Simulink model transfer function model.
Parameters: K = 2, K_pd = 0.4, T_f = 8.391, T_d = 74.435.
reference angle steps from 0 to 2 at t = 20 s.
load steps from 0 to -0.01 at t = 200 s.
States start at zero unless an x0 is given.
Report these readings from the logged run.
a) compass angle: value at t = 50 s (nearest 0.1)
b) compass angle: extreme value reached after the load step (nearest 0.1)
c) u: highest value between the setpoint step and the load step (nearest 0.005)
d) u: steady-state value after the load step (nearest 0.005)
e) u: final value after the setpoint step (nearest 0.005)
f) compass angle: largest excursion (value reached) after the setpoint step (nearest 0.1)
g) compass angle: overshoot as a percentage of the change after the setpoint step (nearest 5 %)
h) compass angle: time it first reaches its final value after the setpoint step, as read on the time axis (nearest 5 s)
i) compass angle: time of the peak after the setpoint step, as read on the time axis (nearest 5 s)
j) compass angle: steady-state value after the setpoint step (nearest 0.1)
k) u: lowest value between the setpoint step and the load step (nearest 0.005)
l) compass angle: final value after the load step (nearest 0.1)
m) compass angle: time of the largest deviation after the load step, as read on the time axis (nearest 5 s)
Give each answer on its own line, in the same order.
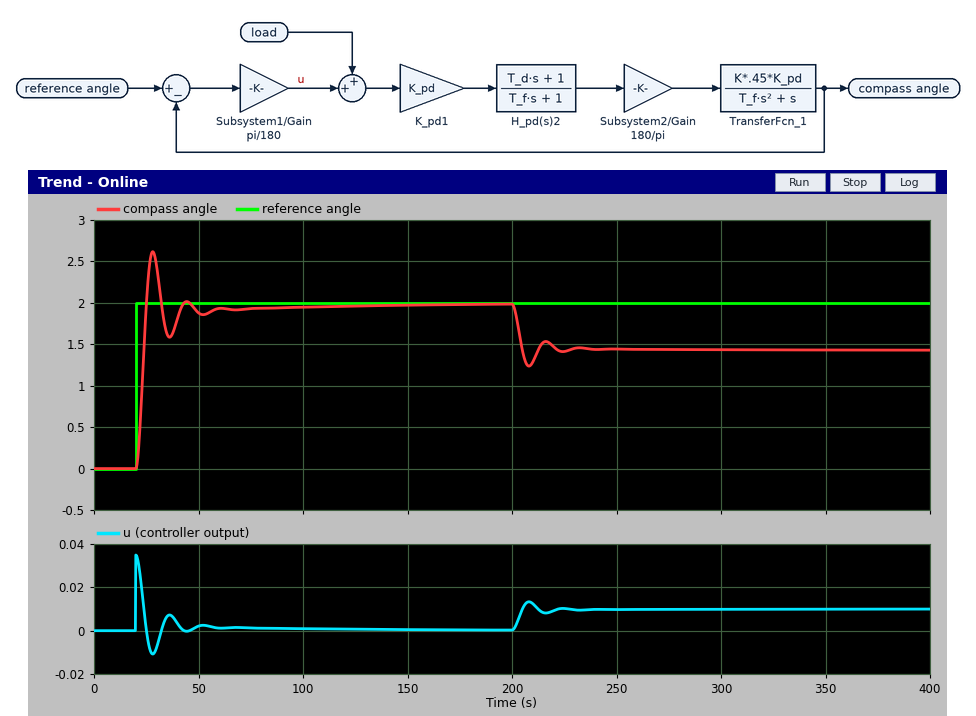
1.9
1.2
0.035
0.010
0.000
2.6
30 %
25 s
30 s
2.0
-0.010
1.4
210 s
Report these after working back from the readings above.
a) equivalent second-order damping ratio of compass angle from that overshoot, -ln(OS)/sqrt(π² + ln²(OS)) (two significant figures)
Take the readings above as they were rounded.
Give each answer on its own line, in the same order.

0.36
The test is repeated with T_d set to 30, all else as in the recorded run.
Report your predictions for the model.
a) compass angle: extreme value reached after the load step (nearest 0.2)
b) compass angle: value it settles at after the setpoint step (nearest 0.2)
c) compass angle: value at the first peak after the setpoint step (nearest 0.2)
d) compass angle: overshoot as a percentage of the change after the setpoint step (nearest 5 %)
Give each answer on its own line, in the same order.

1.4
2.0
2.2
15 %
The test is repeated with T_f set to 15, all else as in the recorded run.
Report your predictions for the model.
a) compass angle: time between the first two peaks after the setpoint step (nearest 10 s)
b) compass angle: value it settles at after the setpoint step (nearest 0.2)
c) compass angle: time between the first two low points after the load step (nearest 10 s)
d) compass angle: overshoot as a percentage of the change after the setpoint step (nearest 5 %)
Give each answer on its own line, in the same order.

30 s
2.0
30 s
35 %
